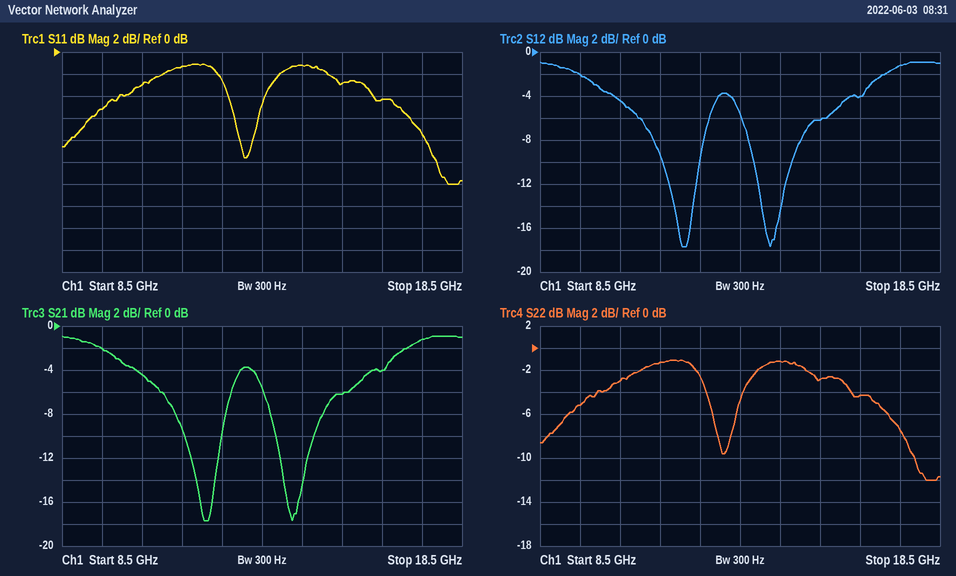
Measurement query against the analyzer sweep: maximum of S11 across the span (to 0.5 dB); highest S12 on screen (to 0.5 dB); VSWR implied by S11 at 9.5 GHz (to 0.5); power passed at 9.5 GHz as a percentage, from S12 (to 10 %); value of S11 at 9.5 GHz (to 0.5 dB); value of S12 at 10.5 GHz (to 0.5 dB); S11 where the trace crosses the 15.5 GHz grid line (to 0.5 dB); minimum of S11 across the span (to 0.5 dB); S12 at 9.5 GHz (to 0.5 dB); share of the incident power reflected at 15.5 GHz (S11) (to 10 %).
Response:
-1.0 dB
-1.0 dB
3.5
60 %
-5.0 dB
-4.5 dB
-3.0 dB
-12.0 dB
-2.0 dB
50 %
